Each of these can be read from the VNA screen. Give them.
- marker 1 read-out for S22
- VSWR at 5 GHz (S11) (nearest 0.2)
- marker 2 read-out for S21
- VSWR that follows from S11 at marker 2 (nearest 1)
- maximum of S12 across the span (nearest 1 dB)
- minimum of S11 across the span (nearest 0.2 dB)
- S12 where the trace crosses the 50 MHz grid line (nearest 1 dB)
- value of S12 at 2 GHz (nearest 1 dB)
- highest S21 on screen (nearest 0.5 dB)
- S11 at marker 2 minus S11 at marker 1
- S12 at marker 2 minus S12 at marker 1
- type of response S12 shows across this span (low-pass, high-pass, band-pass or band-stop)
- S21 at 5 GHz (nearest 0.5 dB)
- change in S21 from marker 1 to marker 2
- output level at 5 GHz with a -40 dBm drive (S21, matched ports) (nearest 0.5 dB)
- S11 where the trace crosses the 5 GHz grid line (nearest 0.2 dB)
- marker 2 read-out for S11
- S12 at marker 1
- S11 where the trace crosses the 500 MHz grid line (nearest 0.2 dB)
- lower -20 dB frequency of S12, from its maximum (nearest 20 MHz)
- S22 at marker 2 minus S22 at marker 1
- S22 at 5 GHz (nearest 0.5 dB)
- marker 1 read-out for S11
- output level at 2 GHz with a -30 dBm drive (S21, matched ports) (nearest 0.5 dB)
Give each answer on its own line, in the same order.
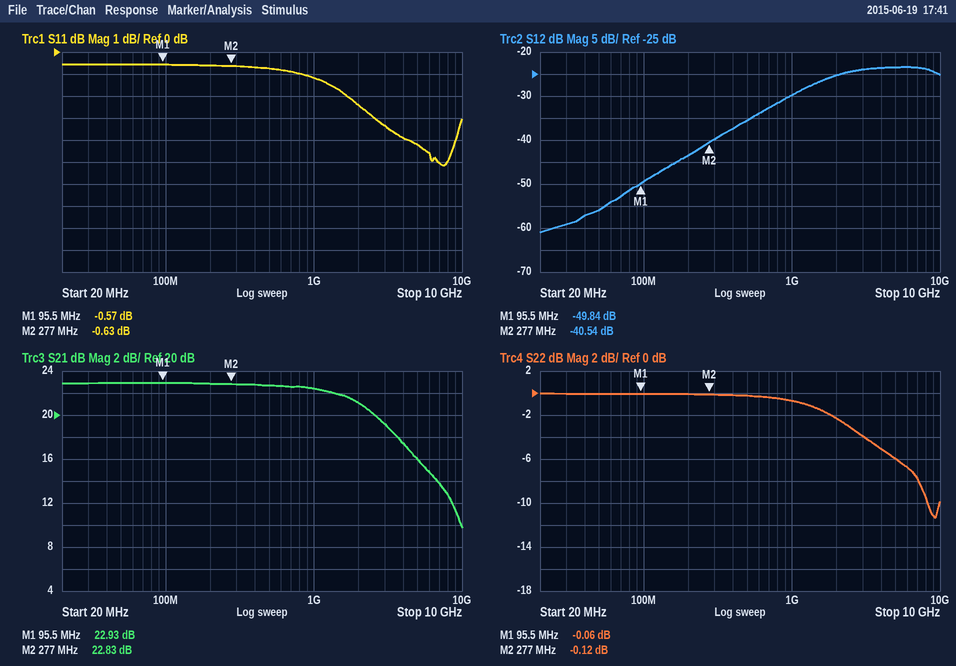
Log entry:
-0.06 dB
4.2
22.83 dB
28
-23 dB
-5.2 dB
-56 dB
-25 dB
23.0 dB
-0.06 dB
9.30 dB
high-pass
16.0 dB
-0.10 dB
-24.0 dBm
-4.2 dB
-0.63 dB
-49.84 dB
-0.8 dB
200 MHz
-0.06 dB
-6.0 dB
-0.57 dB
-9.0 dBm
